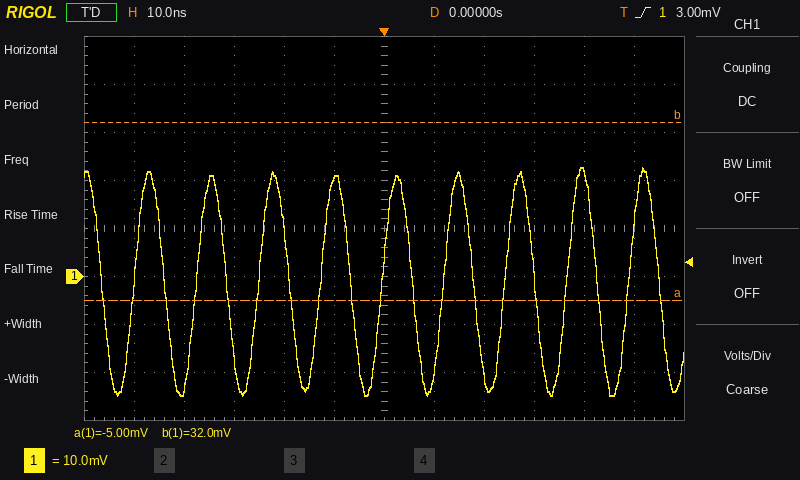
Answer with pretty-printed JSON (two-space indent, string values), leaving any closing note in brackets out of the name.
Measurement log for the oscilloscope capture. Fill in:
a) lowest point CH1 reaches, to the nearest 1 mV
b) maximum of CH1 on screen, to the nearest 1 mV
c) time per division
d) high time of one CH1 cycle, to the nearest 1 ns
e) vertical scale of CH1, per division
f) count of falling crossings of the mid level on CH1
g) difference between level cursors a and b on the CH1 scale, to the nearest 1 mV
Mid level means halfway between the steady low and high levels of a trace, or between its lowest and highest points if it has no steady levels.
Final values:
{
  "lowest point CH1 reaches, to the nearest 1 mV": "-25 mV",
  "maximum of CH1 on screen, to the nearest 1 mV": "23 mV",
  "time per division": "10 ns",
  "high time of one CH1 cycle, to the nearest 1 ns": "6 ns",
  "vertical scale of CH1, per division": "10 mV",
  "count of falling crossings of the mid level on CH1": "10",
  "difference between level cursors a and b on the CH1 scale, to the nearest 1 mV": "37 mV"
}
